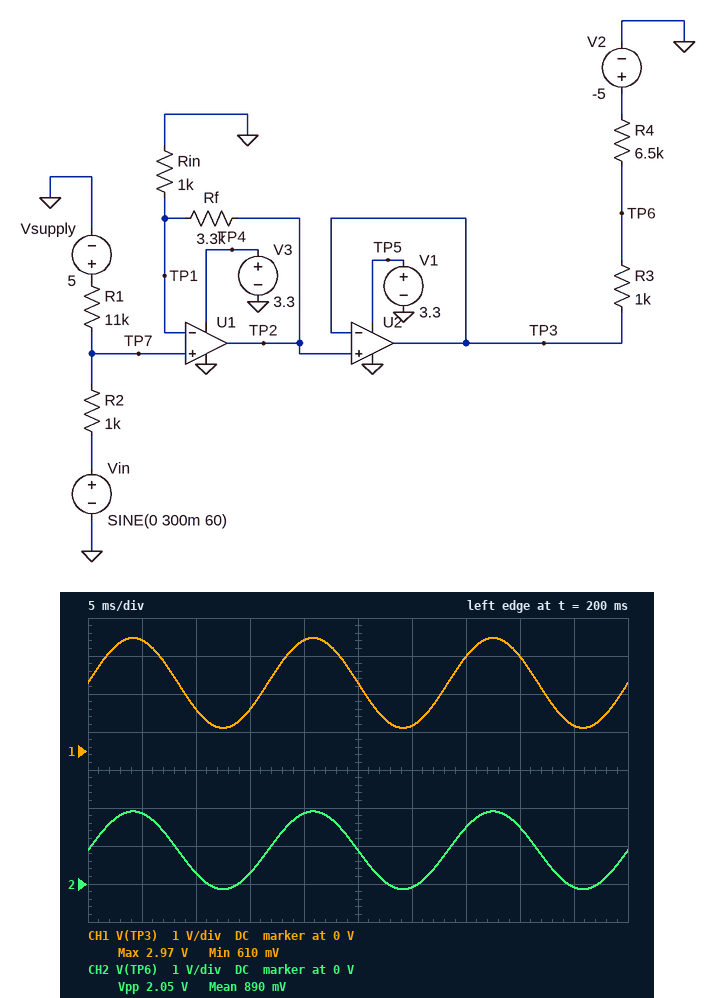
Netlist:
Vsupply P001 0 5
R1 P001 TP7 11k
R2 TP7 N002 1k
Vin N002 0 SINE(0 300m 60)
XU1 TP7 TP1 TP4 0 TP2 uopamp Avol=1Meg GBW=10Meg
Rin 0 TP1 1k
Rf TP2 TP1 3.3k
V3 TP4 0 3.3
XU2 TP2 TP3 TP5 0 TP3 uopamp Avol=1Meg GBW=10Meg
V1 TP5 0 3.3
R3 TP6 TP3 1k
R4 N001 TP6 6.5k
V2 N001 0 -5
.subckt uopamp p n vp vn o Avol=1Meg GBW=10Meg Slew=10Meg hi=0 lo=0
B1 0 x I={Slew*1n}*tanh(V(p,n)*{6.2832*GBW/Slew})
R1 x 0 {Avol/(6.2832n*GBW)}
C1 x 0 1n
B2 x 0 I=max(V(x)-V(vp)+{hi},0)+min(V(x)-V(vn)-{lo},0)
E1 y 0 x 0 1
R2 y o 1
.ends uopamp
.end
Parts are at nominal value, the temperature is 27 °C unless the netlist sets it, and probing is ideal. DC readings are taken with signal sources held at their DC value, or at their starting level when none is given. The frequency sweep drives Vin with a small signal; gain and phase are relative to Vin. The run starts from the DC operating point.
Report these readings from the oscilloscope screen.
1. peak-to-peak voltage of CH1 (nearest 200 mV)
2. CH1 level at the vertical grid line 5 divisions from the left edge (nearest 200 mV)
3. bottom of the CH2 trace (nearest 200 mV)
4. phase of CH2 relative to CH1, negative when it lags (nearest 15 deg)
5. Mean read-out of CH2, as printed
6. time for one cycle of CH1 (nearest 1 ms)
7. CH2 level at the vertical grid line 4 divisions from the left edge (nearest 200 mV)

2.4 V
1.8 V
-200 mV
0 deg
890 mV
17 ms
1.8 V
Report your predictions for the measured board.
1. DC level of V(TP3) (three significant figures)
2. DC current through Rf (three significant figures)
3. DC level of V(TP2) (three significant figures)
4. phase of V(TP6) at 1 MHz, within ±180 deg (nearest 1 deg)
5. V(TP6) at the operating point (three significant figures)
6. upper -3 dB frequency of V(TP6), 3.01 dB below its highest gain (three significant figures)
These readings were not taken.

1.79 V
417 µA
1.79 V
-29 deg
886 mV
2.21 MHz
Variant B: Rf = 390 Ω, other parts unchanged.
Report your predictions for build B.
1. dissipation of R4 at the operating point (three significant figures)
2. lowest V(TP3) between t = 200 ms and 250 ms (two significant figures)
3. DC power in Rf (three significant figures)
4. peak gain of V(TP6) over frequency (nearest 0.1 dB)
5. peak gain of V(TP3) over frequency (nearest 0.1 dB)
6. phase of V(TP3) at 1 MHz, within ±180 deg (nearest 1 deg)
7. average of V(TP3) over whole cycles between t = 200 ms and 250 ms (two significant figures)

3.60 mW
200 mV
67.7 µW
0.9 dB
2.1 dB
-14 deg
580 mV
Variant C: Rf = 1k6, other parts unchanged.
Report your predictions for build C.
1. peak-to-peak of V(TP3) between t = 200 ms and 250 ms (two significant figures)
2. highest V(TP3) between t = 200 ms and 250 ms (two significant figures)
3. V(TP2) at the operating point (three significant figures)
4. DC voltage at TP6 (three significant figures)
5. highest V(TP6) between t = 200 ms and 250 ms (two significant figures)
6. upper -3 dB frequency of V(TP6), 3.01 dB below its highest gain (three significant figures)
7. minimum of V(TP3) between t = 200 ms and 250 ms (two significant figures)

1.4 V
1.8 V
1.08 V
272 mV
890 mV
3.42 MHz
370 mV
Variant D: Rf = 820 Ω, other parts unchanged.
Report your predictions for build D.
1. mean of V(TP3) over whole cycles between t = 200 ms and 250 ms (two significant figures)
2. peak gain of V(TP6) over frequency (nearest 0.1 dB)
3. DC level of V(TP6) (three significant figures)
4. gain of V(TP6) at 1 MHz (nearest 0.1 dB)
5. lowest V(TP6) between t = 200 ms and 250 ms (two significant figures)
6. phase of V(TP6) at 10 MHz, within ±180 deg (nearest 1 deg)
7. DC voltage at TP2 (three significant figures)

760 mV
3.2 dB
-9.45 mV
3.0 dB
-440 mV
-106 deg
758 mV
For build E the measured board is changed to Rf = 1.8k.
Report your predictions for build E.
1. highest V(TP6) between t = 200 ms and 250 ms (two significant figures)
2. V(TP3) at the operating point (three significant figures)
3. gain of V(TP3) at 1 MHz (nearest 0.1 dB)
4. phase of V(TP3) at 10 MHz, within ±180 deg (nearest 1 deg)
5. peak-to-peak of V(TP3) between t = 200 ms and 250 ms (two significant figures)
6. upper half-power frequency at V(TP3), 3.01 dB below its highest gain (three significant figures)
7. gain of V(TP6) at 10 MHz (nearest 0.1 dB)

1.0 V
1.17 V
7.8 dB
-115 deg
1.5 V
3.22 MHz
-5.5 dB
